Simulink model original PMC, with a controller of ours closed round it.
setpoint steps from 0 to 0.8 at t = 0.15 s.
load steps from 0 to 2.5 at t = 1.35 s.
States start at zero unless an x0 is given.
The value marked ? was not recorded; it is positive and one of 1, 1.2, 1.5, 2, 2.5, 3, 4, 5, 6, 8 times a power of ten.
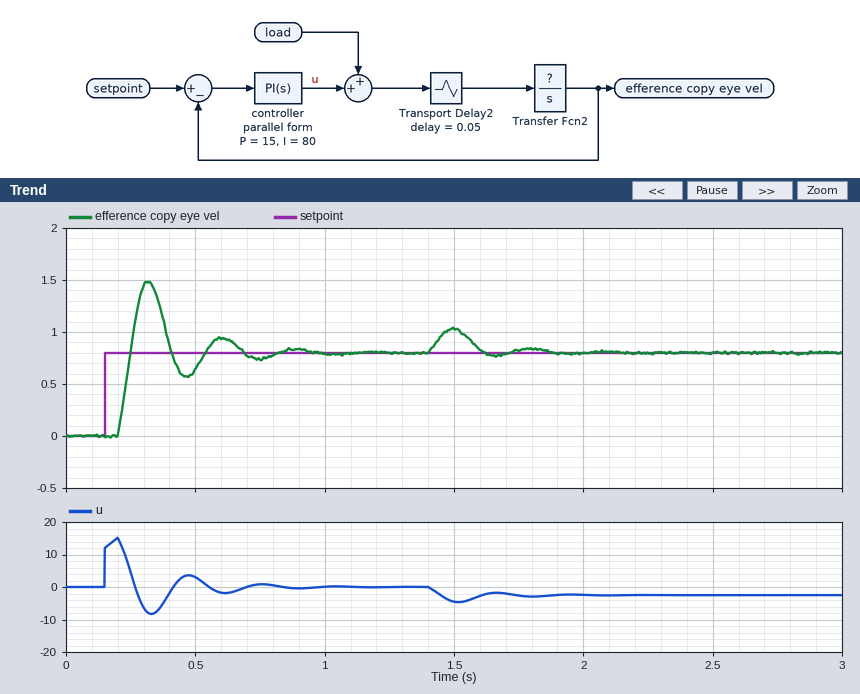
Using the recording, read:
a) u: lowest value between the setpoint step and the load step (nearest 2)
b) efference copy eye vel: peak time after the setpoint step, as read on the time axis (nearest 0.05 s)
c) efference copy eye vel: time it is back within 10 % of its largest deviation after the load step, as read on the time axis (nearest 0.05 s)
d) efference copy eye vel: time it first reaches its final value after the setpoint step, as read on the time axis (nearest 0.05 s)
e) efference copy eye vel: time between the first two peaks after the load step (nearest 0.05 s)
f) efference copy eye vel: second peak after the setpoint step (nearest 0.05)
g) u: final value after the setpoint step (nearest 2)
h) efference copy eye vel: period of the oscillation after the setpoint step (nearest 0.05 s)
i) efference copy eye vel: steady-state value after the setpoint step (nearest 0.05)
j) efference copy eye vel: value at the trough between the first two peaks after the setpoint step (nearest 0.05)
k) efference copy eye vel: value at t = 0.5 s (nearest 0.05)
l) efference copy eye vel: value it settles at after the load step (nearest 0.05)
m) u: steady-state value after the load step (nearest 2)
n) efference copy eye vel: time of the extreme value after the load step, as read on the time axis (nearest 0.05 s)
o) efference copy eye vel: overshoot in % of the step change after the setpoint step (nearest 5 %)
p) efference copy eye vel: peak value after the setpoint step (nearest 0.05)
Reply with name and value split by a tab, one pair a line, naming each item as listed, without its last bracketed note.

u: lowest value between the setpoint step and the load step	-8
efference copy eye vel: peak time after the setpoint step, as read on the time axis	0.30 s
efference copy eye vel: time it is back within 10 % of its largest deviation after the load step, as read on the time axis	1.85 s
efference copy eye vel: time it first reaches its final value after the setpoint step, as read on the time axis	0.25 s
efference copy eye vel: time between the first two peaks after the load step	0.30 s
efference copy eye vel: second peak after the setpoint step	0.95
u: final value after the setpoint step	0
efference copy eye vel: period of the oscillation after the setpoint step	0.30 s
efference copy eye vel: steady-state value after the setpoint step	0.80
efference copy eye vel: value at the trough between the first two peaks after the setpoint step	0.55
efference copy eye vel: value at t = 0.5 s	0.65
efference copy eye vel: value it settles at after the load step	0.80
u: steady-state value after the load step	-2
efference copy eye vel: time of the extreme value after the load step, as read on the time axis	1.50 s
efference copy eye vel: overshoot in % of the step change after the setpoint step	85 %
efference copy eye vel: peak value after the setpoint step	1.50
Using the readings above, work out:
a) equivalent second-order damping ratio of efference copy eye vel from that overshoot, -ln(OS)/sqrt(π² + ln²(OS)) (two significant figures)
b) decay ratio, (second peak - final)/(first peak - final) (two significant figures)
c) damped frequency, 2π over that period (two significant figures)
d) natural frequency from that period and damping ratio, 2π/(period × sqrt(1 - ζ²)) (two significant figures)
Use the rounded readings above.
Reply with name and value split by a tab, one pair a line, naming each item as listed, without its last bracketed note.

equivalent second-order damping ratio of efference copy eye vel from that overshoot, -ln(OS)/sqrt(π² + ln²(OS))	0.052
decay ratio, (second peak - final)/(first peak - final)	0.21
damped frequency, 2π over that period	21 rad/s
natural frequency from that period and damping ratio, 2π/(period × sqrt(1 - ζ²))	21 rad/s
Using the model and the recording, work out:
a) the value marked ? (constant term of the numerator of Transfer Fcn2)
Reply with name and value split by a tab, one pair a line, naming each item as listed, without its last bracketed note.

the value marked ?	1.2
